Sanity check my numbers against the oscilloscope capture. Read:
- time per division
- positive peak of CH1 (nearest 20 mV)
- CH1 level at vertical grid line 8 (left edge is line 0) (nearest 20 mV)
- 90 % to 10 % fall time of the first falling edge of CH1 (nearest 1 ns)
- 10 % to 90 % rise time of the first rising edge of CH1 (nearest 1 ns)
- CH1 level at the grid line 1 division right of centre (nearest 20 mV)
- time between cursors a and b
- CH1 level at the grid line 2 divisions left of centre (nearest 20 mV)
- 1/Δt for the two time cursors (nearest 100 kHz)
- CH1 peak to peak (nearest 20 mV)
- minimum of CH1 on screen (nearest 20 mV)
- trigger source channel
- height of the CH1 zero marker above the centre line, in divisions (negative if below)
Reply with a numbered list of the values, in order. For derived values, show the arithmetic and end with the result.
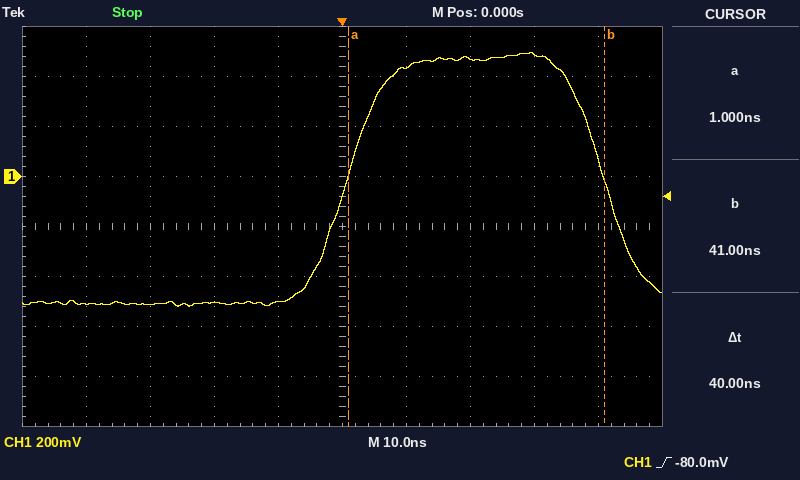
1. 10 ns
2. 500 mV
3. 480 mV
4. 12 ns
5. 12 ns
6. 440 mV
7. 40 ns
8. -500 mV
9. 1 / 40 ns ≈ 25.0 MHz
10. 500 mV − (-520 mV) = 1.02 V
11. -520 mV
12. CH1
13. +1.0 div
